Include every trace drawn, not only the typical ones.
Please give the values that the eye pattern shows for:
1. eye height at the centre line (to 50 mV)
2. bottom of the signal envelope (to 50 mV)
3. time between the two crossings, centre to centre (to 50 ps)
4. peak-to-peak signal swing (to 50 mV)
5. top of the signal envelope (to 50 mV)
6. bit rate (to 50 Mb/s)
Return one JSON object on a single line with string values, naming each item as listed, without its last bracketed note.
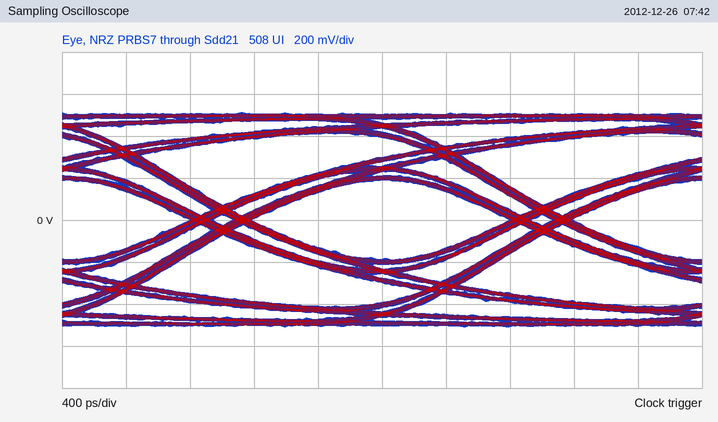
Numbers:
{"eye height at the centre line": "400 mV", "bottom of the signal envelope": "-500 mV", "time between the two crossings, centre to centre": "2.00 ns", "peak-to-peak signal swing": "1.00 V", "top of the signal envelope": "500 mV", "bit rate": "500 Mb/s"}
